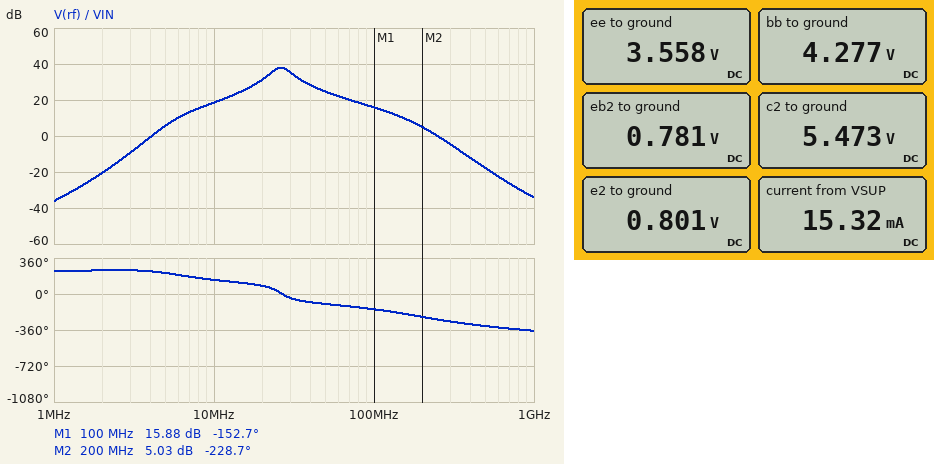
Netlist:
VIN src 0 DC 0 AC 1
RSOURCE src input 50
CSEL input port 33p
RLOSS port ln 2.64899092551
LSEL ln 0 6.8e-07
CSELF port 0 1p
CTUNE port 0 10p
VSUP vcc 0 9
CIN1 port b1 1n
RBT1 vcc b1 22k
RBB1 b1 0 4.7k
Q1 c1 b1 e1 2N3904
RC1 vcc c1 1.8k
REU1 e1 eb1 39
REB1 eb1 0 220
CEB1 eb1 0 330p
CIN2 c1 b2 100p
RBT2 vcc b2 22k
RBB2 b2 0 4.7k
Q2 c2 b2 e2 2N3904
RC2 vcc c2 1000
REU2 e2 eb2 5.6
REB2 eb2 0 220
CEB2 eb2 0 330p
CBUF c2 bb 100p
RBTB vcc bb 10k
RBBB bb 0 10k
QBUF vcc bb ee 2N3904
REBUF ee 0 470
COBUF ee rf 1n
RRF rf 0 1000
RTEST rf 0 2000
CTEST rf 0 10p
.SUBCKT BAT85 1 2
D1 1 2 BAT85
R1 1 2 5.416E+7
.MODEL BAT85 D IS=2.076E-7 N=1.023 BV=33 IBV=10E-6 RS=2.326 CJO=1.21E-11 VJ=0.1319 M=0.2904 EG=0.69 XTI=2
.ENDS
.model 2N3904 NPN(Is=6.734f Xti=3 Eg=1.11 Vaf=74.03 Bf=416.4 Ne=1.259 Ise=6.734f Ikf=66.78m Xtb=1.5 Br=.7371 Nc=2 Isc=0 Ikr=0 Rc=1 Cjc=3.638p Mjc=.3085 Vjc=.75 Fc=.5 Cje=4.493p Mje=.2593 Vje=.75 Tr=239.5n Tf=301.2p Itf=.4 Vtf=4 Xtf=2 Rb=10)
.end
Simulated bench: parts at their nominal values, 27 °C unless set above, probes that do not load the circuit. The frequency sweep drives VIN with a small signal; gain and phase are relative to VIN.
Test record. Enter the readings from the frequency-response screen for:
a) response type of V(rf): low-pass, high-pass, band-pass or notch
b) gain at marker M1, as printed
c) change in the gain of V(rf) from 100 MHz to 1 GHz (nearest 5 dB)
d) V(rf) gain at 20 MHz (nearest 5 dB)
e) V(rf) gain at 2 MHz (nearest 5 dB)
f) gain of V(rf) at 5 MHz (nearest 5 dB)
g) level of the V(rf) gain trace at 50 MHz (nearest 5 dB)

band-pass
15.88 dB
-50 dB
30 dB
-20 dB
5 dB
25 dB
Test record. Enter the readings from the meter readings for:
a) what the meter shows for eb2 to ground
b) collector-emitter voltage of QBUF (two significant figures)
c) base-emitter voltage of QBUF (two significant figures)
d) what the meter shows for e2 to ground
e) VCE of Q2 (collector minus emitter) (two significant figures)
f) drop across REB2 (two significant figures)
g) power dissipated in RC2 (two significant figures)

0.781 V
5.4 V
720 mV
0.801 V
4.7 V
780 mV
12 mW
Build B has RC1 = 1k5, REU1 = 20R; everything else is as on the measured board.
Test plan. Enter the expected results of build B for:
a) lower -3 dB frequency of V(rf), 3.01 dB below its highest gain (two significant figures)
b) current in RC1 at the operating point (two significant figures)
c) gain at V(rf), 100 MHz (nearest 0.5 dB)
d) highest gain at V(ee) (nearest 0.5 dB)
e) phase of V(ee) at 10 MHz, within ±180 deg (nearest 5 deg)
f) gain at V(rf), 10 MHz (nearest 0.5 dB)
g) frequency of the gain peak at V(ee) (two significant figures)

22 MHz
3.3 mA
19.0 dB
42.0 dB
155 deg
20.5 dB
25 MHz
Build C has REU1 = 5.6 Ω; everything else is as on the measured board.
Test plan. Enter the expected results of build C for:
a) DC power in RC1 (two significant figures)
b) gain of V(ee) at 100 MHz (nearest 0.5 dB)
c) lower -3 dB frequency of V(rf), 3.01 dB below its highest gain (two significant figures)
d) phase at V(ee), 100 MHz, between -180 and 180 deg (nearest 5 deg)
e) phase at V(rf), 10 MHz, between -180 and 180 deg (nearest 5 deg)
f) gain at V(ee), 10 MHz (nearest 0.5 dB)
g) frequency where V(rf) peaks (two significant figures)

22 mW
22.5 dB
22 MHz
-145 deg
165 deg
22.0 dB
24 MHz
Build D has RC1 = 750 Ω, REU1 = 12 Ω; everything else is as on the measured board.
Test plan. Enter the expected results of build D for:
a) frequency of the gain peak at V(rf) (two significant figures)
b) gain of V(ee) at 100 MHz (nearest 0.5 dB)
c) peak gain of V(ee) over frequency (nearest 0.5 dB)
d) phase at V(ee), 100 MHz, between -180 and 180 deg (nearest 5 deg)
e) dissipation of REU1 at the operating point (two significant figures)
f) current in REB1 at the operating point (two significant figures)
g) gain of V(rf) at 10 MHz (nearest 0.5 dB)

25 MHz
21.0 dB
46.5 dB
-145 deg
140 µW
3.5 mA
21.5 dB
